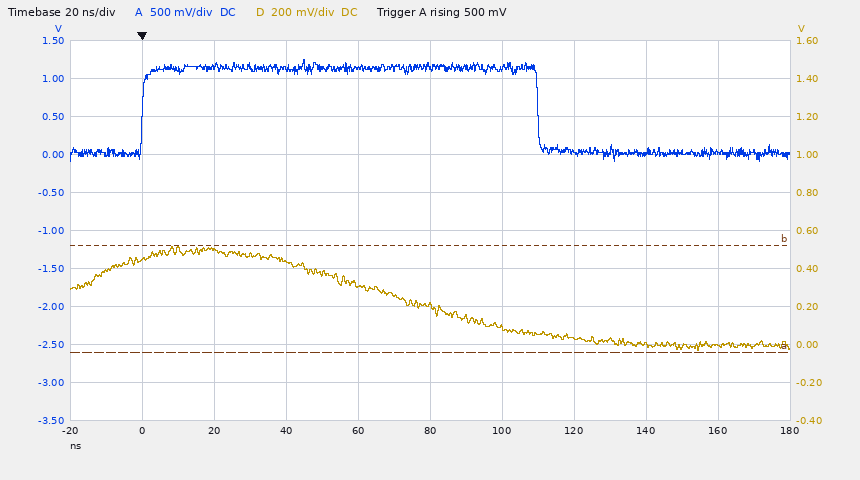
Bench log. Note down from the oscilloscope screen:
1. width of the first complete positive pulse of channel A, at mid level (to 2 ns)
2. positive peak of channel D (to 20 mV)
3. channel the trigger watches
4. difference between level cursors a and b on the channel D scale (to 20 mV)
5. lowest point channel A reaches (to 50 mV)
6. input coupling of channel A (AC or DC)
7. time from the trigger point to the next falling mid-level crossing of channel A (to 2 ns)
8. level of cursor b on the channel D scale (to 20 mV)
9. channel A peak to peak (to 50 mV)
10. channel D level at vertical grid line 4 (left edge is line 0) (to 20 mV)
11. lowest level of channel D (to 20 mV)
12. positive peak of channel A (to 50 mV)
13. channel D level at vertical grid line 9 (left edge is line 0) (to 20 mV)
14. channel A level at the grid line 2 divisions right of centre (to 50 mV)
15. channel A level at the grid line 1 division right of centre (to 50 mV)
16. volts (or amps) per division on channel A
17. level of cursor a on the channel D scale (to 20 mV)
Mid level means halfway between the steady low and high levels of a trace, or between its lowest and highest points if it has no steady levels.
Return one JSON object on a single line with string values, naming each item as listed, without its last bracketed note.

{"width of the first complete positive pulse of channel A, at mid level": "110 ns", "positive peak of channel D": "520 mV", "channel the trigger watches": "channel A", "difference between level cursors a and b on the channel D scale": "560 mV", "lowest point channel A reaches": "-100 mV", "input coupling of channel A": "DC", "time from the trigger point to the next falling mid-level crossing of channel A": "110 ns", "level of cursor b on the channel D scale": "520 mV", "channel A peak to peak": "1.35 V", "channel D level at vertical grid line 4 (left edge is line 0)": "320 mV", "lowest level of channel D": "-40 mV", "positive peak of channel A": "1.25 V", "channel D level at vertical grid line 9 (left edge is line 0)": "0 mV", "channel A level at the grid line 2 divisions right of centre": "50 mV", "channel A level at the grid line 1 division right of centre": "1.15 V", "volts (or amps) per division on channel A": "500 mV", "level of cursor a on the channel D scale": "-40 mV"}
